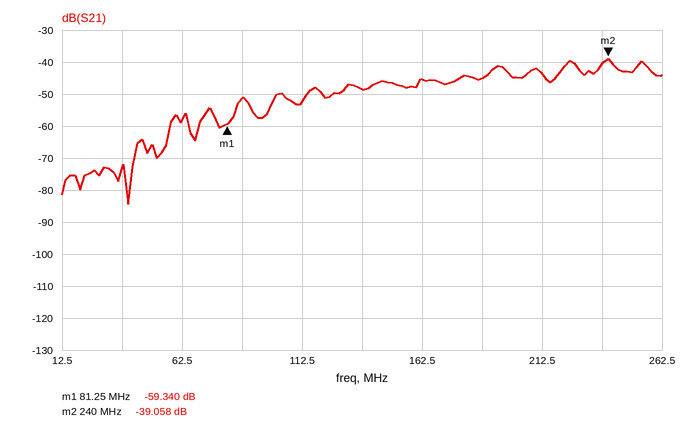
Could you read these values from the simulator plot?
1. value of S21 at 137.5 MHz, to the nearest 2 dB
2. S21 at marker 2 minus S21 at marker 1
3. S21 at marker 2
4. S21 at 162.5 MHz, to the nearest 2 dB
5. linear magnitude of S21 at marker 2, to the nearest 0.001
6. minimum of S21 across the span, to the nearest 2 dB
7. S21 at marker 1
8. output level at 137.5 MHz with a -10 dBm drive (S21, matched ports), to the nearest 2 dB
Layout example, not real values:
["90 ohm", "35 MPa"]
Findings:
["-48 dB", "20.282 dB", "-39.058 dB", "-46 dB", "0.011", "-84 dB", "-59.340 dB", "-58 dBm"]
